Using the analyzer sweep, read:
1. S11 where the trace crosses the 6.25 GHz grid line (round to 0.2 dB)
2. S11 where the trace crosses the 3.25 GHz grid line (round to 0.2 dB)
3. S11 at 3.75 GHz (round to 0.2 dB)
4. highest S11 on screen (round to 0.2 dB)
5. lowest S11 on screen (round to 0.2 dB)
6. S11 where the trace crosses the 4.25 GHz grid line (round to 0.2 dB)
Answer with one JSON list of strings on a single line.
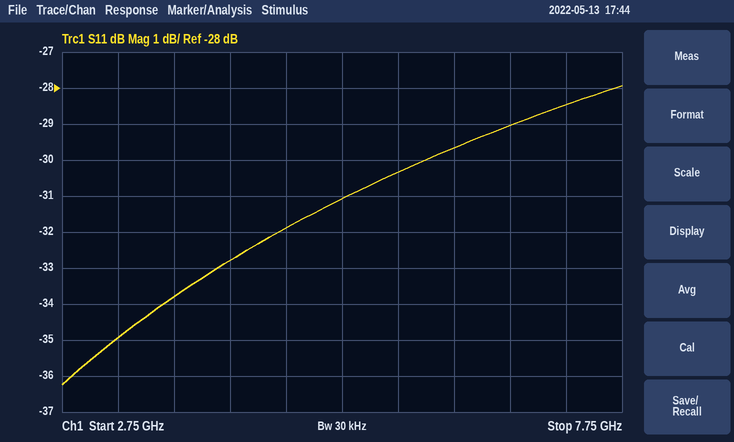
["-29.6 dB", "-35.0 dB", "-33.8 dB", "-28.0 dB", "-36.2 dB", "-32.8 dB"]
